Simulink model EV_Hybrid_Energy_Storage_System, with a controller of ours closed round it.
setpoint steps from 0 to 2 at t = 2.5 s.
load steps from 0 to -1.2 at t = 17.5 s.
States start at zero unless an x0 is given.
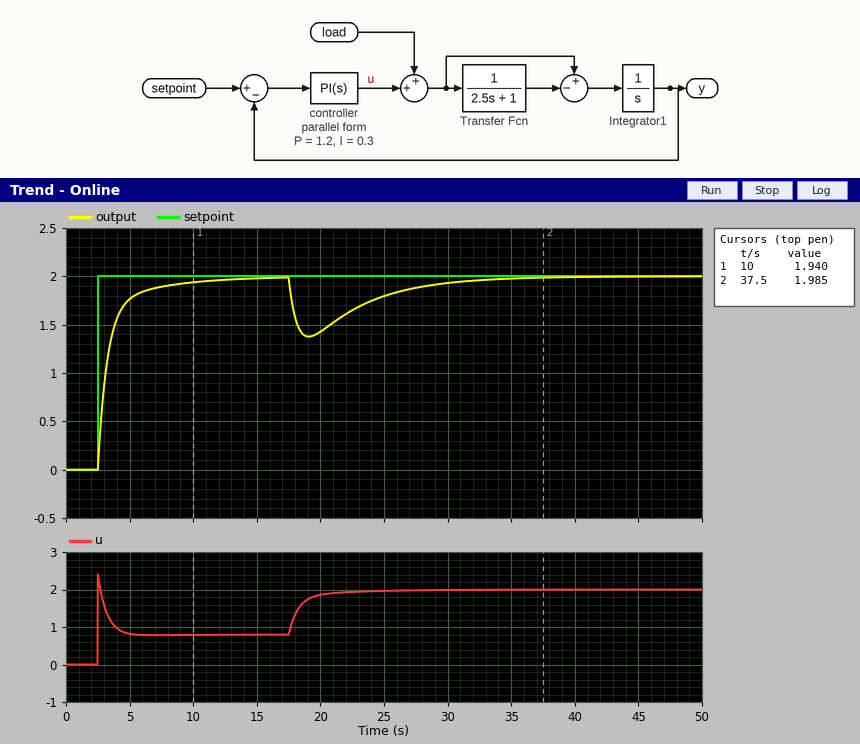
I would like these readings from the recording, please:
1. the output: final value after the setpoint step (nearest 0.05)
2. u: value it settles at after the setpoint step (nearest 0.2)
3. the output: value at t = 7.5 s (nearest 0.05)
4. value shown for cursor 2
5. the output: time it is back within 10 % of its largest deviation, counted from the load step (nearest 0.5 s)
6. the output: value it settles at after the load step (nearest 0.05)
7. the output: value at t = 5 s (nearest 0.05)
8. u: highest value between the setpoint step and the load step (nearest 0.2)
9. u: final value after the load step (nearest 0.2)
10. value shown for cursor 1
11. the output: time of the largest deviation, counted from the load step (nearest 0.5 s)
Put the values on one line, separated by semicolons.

2.00; 0.8; 1.90; 1.985; 13.0 s; 2.00; 1.75; 2.4; 2.0; 1.940; 1.5 s
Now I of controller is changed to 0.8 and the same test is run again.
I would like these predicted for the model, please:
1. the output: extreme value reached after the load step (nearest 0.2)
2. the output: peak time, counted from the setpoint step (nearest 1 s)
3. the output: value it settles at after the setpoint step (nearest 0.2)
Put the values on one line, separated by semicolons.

1.4; 3 s; 2.0
